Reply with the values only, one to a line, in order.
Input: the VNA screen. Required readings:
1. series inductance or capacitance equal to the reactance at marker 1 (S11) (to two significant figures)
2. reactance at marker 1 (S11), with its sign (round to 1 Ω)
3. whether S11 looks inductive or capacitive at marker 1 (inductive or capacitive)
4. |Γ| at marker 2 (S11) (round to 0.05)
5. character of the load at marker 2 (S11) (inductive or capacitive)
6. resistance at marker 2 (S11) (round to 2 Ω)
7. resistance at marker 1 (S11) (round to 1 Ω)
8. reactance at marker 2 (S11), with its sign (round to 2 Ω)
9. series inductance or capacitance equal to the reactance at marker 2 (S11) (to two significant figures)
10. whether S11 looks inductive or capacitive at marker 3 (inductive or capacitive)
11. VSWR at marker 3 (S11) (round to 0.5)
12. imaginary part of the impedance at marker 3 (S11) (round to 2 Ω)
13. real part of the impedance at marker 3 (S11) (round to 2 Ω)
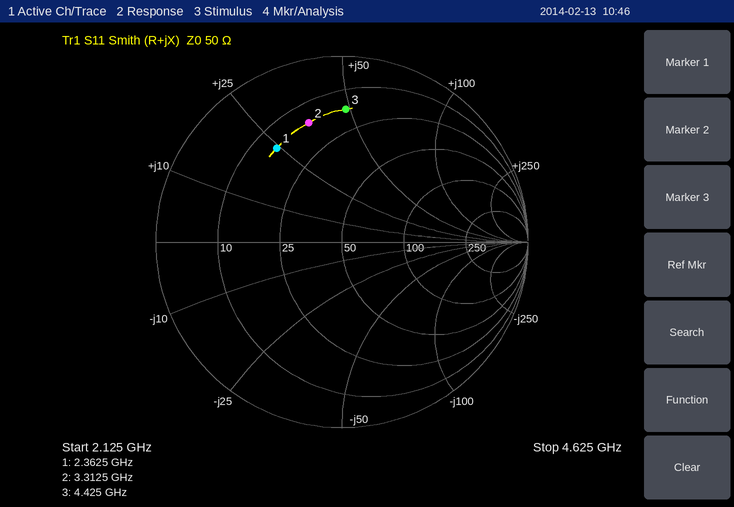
1.6 nH
+24 Ω
inductive
0.65
inductive
16 Ω
15 Ω
+36 Ω
1.7 nH
inductive
6.0
+48 Ω
16 Ω
